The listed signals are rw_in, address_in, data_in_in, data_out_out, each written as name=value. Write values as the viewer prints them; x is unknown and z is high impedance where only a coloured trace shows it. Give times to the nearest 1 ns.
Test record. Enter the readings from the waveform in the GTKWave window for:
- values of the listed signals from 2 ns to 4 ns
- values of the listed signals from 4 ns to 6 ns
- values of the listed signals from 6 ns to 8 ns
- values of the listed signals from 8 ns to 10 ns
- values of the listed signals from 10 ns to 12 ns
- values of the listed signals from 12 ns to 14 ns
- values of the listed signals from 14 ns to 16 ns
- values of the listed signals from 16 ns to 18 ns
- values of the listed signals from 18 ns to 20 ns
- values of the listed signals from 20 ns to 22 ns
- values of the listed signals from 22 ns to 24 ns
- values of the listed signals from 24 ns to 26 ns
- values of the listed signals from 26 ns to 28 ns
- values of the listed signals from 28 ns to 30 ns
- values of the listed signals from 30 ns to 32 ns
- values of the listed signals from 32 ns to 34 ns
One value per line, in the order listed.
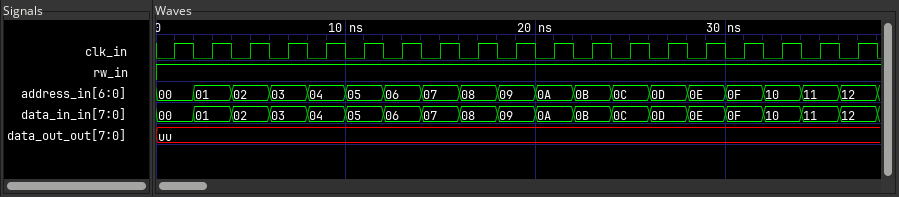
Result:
rw_in=1, address_in=01, data_in_in=01, data_out_out=uu
rw_in=1, address_in=02, data_in_in=02, data_out_out=uu
rw_in=1, address_in=03, data_in_in=03, data_out_out=uu
rw_in=1, address_in=04, data_in_in=04, data_out_out=uu
rw_in=1, address_in=05, data_in_in=05, data_out_out=uu
rw_in=1, address_in=06, data_in_in=06, data_out_out=uu
rw_in=1, address_in=07, data_in_in=07, data_out_out=uu
rw_in=1, address_in=08, data_in_in=08, data_out_out=uu
rw_in=1, address_in=09, data_in_in=09, data_out_out=uu
rw_in=1, address_in=0A, data_in_in=0A, data_out_out=uu
rw_in=1, address_in=0B, data_in_in=0B, data_out_out=uu
rw_in=1, address_in=0C, data_in_in=0C, data_out_out=uu
rw_in=1, address_in=0D, data_in_in=0D, data_out_out=uu
rw_in=1, address_in=0E, data_in_in=0E, data_out_out=uu
rw_in=1, address_in=0F, data_in_in=0F, data_out_out=uu
rw_in=1, address_in=10, data_in_in=10, data_out_out=uu
